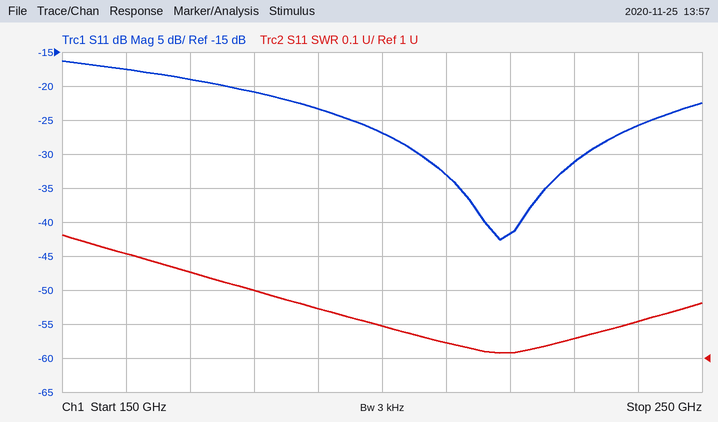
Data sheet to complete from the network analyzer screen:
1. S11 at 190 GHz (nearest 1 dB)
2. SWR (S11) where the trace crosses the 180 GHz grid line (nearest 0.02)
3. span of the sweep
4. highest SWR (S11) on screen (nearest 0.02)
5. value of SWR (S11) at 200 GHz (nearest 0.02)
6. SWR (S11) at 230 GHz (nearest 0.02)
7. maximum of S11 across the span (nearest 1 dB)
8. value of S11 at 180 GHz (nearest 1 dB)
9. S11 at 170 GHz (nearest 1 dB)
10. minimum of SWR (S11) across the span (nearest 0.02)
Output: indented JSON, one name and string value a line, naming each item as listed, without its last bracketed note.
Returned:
{
  "S11 at 190 GHz": "-23 dB",
  "SWR (S11) where the trace crosses the 180 GHz grid line": "1.20",
  "span of the sweep": "100 GHz",
  "highest SWR (S11) on screen": "1.36",
  "value of SWR (S11) at 200 GHz": "1.10",
  "SWR (S11) at 230 GHz": "1.06",
  "maximum of S11 across the span": "-16 dB",
  "value of S11 at 180 GHz": "-21 dB",
  "S11 at 170 GHz": "-19 dB",
  "minimum of SWR (S11) across the span": "1.02"
}
